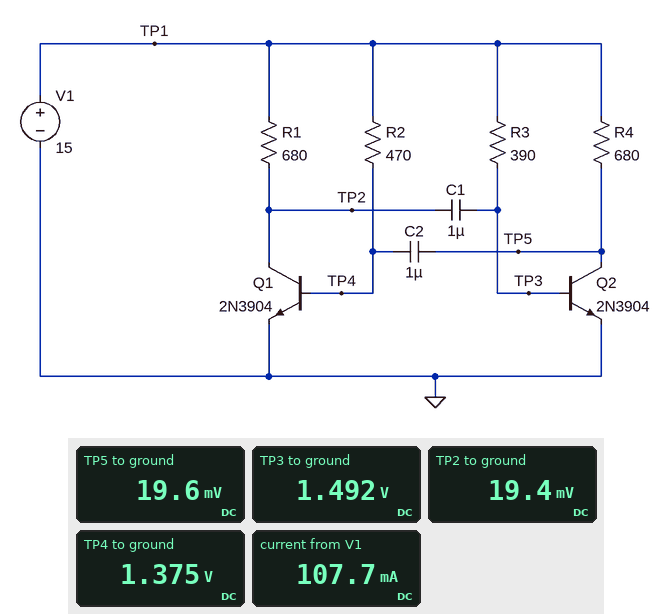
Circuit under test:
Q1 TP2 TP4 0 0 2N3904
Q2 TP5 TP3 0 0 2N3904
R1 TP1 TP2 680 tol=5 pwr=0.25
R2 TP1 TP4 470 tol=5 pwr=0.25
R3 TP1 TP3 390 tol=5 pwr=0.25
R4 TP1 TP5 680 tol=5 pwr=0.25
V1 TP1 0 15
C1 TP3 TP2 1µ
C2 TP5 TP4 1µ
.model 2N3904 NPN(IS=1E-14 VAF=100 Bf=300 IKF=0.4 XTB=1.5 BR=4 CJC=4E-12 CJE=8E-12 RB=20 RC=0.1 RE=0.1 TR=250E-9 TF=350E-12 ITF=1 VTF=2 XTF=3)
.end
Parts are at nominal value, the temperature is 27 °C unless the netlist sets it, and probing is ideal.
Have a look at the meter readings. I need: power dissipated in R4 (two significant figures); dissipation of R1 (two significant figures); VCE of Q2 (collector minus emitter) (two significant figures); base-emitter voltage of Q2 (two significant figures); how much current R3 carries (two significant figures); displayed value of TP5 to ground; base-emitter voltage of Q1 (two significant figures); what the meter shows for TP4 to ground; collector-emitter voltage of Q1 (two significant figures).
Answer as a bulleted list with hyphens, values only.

- 330 mW
- 330 mW
- 20 mV
- 1.5 V
- 35 mA
- 19.6 mV
- 1.4 V
- 1.375 V
- 19 mV
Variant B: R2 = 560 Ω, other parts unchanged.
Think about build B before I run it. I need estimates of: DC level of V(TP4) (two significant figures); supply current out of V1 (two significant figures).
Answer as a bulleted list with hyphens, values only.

- 1.3 V
- 100 mA
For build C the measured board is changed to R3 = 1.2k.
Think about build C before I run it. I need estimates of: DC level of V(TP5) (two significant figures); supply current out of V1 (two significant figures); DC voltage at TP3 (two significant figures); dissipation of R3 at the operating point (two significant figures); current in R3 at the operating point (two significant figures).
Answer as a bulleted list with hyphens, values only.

- 22 mV
- 85 mA
- 1.0 V
- 160 mW
- 12 mA
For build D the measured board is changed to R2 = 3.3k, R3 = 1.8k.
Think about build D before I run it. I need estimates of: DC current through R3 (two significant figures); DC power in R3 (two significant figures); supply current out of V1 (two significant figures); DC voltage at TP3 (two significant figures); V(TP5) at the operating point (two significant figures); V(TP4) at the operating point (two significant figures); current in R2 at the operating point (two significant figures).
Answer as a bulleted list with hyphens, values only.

- 7.8 mA
- 110 mW
- 56 mA
- 920 mV
- 25 mV
- 840 mV
- 4.3 mA
